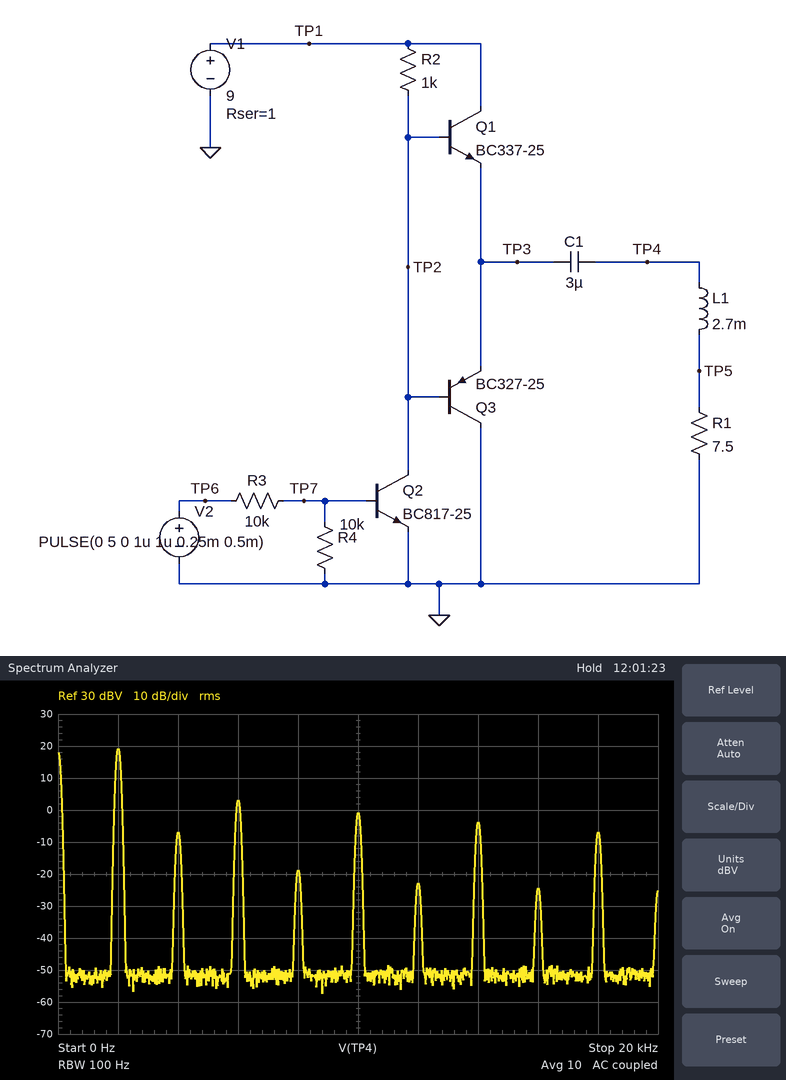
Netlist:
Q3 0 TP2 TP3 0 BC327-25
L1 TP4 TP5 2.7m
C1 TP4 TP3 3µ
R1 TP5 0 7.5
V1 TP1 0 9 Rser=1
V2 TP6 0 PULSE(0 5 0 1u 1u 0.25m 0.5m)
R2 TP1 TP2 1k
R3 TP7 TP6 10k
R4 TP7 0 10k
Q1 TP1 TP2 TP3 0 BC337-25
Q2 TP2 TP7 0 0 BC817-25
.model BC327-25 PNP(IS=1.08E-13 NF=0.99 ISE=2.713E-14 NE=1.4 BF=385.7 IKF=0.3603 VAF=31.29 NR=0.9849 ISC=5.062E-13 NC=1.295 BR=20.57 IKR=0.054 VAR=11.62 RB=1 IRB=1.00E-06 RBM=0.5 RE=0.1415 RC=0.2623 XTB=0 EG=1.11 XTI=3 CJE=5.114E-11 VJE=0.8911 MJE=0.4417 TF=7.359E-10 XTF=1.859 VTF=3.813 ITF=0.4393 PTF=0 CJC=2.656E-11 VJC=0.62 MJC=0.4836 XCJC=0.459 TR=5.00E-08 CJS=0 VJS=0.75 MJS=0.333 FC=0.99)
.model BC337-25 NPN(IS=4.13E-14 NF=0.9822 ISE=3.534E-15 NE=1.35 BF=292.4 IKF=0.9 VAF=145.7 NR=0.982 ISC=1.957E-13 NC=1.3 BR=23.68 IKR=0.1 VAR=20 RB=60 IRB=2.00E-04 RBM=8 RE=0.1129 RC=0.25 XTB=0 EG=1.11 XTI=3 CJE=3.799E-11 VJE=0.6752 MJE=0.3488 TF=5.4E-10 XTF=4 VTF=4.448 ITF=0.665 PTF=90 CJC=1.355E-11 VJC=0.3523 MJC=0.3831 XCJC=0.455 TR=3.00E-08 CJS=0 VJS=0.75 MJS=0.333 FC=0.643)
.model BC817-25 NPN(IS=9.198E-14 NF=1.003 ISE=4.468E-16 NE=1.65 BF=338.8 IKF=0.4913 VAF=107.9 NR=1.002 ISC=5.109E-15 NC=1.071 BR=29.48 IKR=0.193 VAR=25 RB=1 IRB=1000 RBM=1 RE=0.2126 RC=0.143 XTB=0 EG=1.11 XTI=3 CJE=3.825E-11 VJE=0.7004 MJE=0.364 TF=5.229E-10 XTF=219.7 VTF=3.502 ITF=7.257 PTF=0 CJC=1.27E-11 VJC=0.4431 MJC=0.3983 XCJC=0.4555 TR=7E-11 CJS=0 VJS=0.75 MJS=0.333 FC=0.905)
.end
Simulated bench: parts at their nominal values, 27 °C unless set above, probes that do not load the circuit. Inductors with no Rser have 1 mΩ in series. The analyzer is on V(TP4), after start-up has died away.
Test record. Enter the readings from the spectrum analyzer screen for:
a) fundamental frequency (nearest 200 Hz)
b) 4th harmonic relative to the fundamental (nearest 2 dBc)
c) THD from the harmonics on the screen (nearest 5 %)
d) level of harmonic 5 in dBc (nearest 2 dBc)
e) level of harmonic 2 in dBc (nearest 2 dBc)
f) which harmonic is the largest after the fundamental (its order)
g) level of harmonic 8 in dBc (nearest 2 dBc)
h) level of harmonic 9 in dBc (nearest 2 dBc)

2.0 kHz
-38 dBc
20 %
-20 dBc
-26 dBc
3
-44 dBc
-26 dBc
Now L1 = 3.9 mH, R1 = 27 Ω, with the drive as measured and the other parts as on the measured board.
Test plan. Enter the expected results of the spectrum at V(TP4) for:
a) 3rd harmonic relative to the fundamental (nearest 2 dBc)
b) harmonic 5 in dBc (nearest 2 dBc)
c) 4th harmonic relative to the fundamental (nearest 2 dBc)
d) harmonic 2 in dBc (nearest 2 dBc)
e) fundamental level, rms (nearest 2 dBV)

-12 dBc
-16 dBc
-40 dBc
-34 dBc
14 dBV
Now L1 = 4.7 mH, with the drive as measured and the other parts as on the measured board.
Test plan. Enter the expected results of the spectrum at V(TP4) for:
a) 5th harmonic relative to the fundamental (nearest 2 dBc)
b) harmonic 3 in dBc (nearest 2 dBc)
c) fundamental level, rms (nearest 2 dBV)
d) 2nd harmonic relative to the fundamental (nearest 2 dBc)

-18 dBc
-12 dBc
16 dBV
-30 dBc
